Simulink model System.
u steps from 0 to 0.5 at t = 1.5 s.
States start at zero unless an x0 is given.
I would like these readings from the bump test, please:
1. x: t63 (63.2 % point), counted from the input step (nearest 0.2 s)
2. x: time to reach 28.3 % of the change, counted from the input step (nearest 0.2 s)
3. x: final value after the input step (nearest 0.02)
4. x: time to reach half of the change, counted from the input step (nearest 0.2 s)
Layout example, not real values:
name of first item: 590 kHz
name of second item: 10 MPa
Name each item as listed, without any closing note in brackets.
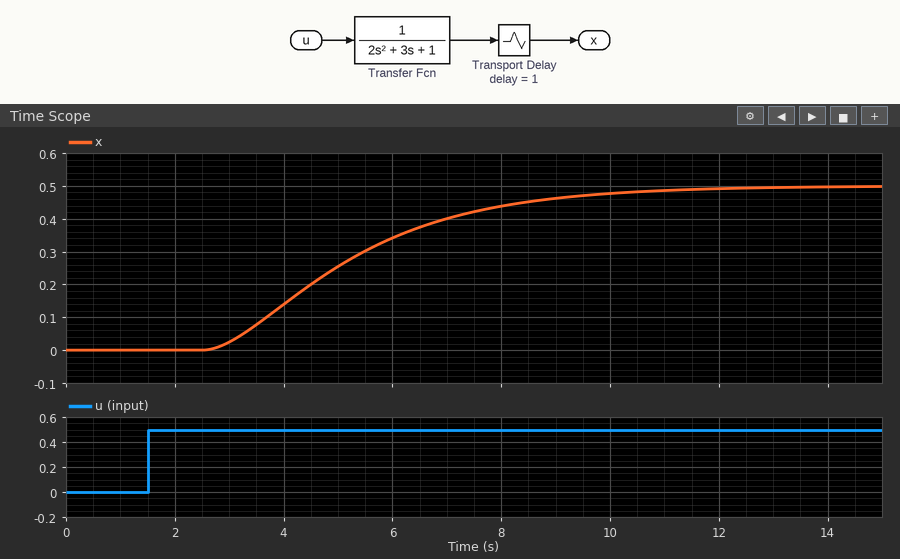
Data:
x: t63 (63.2 % point), counted from the input step: 4.2 s
x: time to reach 28.3 % of the change, counted from the input step: 2.6 s
x: final value after the input step: 0.50
x: time to reach half of the change, counted from the input step: 3.4 s
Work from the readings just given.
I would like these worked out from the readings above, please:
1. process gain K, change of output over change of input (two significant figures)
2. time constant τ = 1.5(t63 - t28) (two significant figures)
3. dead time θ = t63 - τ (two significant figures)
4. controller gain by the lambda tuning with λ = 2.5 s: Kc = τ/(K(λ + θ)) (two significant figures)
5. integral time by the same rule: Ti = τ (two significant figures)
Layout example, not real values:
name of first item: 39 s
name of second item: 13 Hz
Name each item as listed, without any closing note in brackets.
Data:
process gain K, change of output over change of input: 1.0
time constant τ = 1.5(t63 - t28): 2.4 s
dead time θ = t63 - τ: 1.8 s
controller gain by the lambda tuning with λ = 2.5 s: Kc = τ/(K(λ + θ)): 0.56
integral time by the same rule: Ti = τ: 2.4 s
